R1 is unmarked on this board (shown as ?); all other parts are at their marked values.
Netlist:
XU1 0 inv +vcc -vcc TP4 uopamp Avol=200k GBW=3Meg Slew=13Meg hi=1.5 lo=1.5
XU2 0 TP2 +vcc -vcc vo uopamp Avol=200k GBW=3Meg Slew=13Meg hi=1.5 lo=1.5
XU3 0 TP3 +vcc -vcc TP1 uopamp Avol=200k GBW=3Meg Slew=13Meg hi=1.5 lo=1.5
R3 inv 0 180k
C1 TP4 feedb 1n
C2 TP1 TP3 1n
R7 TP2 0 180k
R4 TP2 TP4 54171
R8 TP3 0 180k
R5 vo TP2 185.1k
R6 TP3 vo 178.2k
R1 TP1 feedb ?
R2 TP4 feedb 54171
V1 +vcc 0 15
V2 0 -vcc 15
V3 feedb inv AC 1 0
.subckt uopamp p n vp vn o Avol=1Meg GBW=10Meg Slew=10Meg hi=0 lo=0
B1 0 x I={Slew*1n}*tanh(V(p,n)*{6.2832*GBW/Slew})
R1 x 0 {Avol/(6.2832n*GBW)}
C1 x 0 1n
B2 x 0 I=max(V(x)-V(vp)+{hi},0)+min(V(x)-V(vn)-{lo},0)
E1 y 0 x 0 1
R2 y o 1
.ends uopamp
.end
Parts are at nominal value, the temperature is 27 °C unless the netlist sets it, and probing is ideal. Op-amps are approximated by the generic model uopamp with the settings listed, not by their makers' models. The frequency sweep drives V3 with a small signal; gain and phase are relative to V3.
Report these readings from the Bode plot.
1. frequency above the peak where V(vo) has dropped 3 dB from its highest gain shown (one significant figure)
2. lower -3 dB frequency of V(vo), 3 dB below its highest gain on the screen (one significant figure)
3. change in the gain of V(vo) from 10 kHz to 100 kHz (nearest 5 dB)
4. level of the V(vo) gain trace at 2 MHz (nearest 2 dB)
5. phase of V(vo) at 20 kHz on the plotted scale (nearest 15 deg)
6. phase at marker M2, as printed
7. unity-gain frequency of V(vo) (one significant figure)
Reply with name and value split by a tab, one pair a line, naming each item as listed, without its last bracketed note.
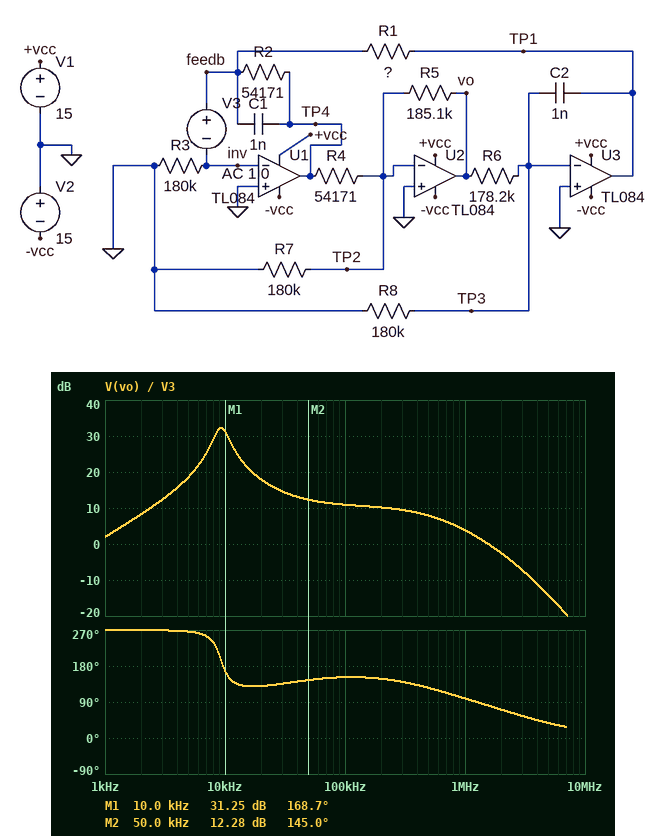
frequency above the peak where V(vo) has dropped 3 dB from its highest gain shown	10 kHz
lower -3 dB frequency of V(vo), 3 dB below its highest gain on the screen	8 kHz
change in the gain of V(vo) from 10 kHz to 100 kHz	-20 dB
level of the V(vo) gain trace at 2 MHz	-2 dB
phase of V(vo) at 20 kHz on the plotted scale	135 deg
phase at marker M2, as printed	145.0 deg
unity-gain frequency of V(vo)	2 MHz
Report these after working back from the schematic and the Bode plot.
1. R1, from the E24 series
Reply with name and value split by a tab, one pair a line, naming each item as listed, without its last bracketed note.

R1, from the E24 series	5.6 kΩ
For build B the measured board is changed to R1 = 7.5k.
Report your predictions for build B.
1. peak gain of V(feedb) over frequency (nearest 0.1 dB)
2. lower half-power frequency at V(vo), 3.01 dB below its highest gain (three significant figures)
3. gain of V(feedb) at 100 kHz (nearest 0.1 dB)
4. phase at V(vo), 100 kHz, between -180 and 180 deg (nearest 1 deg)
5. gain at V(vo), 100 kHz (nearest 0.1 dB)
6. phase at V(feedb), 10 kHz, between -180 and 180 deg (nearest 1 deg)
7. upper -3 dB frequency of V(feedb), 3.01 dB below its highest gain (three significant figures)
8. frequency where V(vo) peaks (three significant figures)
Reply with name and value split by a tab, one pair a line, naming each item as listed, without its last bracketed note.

peak gain of V(feedb) over frequency	0.1 dB
lower half-power frequency at V(vo), 3.01 dB below its highest gain	6.79 kHz
gain of V(feedb) at 100 kHz	-0.1 dB
phase at V(vo), 100 kHz, between -180 and 180 deg	156 deg
gain at V(vo), 100 kHz	10.8 dB
phase at V(feedb), 10 kHz, between -180 and 180 deg	-1 deg
upper -3 dB frequency of V(feedb), 3.01 dB below its highest gain	2.90 MHz
frequency where V(vo) peaks	8.04 kHz
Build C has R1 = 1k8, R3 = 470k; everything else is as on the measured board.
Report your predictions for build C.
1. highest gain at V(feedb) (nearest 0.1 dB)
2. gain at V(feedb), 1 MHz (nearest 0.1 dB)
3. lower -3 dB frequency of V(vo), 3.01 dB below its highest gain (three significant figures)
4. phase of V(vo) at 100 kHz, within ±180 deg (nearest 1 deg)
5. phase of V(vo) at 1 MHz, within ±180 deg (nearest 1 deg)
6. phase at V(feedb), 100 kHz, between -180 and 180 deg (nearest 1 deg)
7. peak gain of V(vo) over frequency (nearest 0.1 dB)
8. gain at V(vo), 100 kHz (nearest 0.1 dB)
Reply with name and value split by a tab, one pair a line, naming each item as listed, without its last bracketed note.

highest gain at V(feedb)	1.0 dB
gain at V(feedb), 1 MHz	-0.7 dB
lower -3 dB frequency of V(vo), 3.01 dB below its highest gain	15.1 kHz
phase of V(vo) at 100 kHz, within ±180 deg	127 deg
phase of V(vo) at 1 MHz, within ±180 deg	96 deg
phase at V(feedb), 100 kHz, between -180 and 180 deg	-2 deg
peak gain of V(vo) over frequency	42.9 dB
gain at V(vo), 100 kHz	13.1 dB
